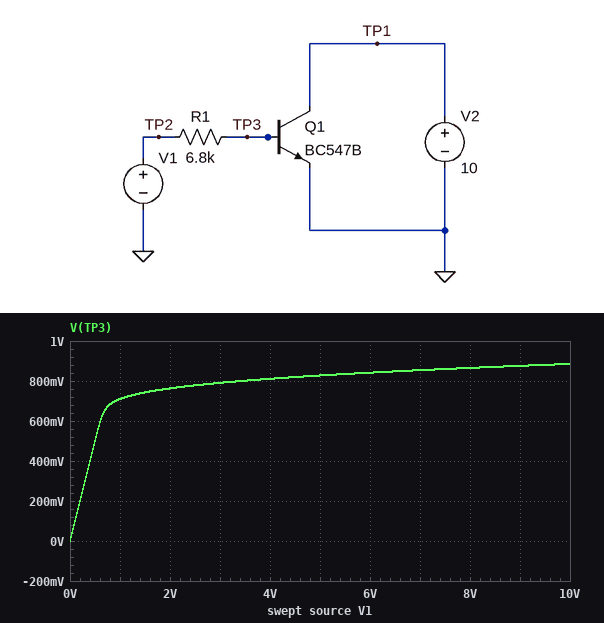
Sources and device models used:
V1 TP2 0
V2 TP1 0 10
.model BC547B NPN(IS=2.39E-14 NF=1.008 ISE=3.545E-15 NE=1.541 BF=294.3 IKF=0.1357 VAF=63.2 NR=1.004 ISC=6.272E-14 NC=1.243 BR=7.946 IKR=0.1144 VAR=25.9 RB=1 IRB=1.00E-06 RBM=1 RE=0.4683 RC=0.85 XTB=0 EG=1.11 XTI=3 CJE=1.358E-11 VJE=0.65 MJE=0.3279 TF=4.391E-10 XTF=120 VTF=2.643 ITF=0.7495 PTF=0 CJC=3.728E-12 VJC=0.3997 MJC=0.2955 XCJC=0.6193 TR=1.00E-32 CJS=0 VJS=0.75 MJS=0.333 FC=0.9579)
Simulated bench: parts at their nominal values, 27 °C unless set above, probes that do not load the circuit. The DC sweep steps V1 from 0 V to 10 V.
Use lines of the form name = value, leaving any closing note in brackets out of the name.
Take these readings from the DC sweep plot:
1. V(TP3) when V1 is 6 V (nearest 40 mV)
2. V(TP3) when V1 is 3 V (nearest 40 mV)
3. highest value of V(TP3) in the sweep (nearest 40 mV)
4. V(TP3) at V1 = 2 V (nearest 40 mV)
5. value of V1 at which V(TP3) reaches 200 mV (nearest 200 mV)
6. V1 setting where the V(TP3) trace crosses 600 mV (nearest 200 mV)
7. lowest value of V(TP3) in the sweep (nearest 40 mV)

V(TP3) when V1 is 6 V = 840 mV
V(TP3) when V1 is 3 V = 800 mV
highest value of V(TP3) in the sweep = 880 mV
V(TP3) at V1 = 2 V = 760 mV
value of V1 at which V(TP3) reaches 200 mV = 200 mV
V1 setting where the V(TP3) trace crosses 600 mV = 600 mV
lowest value of V(TP3) in the sweep = 0 V
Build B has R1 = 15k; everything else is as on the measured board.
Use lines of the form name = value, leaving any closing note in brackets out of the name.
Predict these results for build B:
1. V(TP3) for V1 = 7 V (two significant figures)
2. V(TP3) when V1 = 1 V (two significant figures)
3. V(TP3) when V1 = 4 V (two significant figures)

V(TP3) for V1 = 7 V = 800 mV
V(TP3) when V1 = 1 V = 690 mV
V(TP3) when V1 = 4 V = 770 mV
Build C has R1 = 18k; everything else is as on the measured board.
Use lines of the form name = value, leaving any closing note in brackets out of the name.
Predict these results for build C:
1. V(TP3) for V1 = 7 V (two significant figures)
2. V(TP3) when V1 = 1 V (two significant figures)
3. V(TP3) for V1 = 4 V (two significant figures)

V(TP3) for V1 = 7 V = 790 mV
V(TP3) when V1 = 1 V = 680 mV
V(TP3) for V1 = 4 V = 760 mV
